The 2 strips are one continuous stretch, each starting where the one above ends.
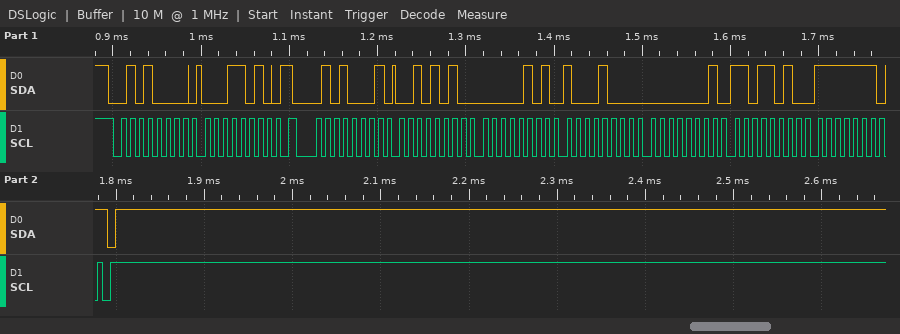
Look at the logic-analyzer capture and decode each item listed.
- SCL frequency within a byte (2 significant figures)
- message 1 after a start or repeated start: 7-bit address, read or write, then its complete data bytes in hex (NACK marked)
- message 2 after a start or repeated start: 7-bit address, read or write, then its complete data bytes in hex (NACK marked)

100 kHz
0x28 write: 1A
0x28 read: 2A 05 88 01 DA FE NACK
